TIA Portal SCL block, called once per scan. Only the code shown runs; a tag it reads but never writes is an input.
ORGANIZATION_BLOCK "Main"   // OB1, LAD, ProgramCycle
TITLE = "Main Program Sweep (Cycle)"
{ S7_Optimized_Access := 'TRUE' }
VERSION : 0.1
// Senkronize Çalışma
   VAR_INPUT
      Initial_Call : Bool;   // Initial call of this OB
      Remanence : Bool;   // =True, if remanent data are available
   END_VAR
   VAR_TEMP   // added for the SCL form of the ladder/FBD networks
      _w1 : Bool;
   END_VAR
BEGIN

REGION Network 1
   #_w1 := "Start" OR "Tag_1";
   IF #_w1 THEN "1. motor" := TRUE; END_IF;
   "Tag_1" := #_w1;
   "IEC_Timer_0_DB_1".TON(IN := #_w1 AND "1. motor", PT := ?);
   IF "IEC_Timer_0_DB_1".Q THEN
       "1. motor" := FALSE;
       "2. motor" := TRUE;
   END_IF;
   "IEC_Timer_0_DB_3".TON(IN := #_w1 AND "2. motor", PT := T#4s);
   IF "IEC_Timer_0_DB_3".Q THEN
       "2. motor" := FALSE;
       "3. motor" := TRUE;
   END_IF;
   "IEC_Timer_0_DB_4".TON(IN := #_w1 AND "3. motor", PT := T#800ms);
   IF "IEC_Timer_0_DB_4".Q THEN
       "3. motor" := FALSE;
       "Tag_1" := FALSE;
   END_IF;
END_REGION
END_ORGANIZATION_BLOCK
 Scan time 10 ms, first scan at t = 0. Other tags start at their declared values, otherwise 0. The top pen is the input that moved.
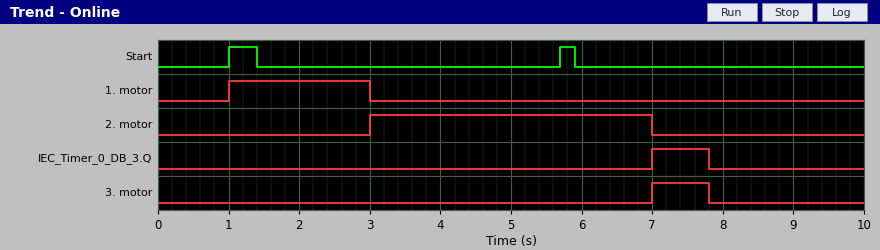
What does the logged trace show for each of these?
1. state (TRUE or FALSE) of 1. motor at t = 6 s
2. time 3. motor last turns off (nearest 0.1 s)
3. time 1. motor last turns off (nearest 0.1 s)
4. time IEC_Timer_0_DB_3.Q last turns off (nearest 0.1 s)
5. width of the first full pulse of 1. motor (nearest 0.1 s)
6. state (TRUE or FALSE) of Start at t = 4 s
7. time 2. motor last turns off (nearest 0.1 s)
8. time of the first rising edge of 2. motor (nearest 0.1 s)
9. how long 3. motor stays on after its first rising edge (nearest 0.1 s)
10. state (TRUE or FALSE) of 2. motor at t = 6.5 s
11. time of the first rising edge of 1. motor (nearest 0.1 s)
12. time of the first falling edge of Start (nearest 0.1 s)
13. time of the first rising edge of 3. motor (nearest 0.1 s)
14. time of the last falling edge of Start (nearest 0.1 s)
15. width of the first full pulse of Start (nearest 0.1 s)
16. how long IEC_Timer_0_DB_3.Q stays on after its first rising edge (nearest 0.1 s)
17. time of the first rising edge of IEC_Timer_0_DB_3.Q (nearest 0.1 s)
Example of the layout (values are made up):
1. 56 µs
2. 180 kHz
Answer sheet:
1. FALSE
2. 7.8 s
3. 3.0 s
4. 7.8 s
5. 2.0 s
6. FALSE
7. 7.0 s
8. 3.0 s
9. 0.8 s
10. TRUE
11. 1.0 s
12. 1.4 s
13. 7.0 s
14. 5.9 s
15. 0.4 s
16. 0.8 s
17. 7.0 s
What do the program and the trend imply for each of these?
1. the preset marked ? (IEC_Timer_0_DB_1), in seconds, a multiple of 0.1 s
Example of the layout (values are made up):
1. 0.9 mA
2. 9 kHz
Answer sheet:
1. 2.0 s
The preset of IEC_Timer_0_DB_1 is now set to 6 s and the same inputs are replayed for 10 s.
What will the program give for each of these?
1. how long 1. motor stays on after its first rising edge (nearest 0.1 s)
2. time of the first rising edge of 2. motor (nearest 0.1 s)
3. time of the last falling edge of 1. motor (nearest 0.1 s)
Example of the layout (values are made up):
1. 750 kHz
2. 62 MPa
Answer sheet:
1. 6.0 s
2. 7.0 s
3. 7.0 s
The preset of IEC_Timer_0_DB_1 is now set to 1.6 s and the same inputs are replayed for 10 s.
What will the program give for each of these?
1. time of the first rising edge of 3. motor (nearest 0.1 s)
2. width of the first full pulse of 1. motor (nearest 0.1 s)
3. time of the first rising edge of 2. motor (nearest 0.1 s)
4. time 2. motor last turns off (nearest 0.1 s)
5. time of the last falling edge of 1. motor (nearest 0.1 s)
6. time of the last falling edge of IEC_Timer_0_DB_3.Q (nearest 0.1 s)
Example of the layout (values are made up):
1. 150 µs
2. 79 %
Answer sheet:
1. 6.6 s
2. 1.6 s
3. 2.6 s
4. 6.6 s
5. 2.6 s
6. 7.4 s
